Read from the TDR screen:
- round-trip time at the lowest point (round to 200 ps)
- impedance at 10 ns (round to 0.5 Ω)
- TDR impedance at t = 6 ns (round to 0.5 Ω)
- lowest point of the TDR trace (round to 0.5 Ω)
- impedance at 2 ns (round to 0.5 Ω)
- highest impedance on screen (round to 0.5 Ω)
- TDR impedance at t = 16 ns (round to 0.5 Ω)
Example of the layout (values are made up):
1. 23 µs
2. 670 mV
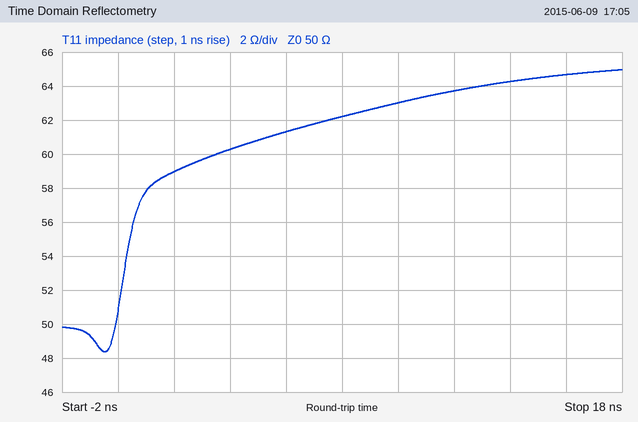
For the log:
1. -400 ps
2. 63.0 Ω
3. 61.5 Ω
4. 48.5 Ω
5. 59.0 Ω
6. 65.0 Ω
7. 64.5 Ω
